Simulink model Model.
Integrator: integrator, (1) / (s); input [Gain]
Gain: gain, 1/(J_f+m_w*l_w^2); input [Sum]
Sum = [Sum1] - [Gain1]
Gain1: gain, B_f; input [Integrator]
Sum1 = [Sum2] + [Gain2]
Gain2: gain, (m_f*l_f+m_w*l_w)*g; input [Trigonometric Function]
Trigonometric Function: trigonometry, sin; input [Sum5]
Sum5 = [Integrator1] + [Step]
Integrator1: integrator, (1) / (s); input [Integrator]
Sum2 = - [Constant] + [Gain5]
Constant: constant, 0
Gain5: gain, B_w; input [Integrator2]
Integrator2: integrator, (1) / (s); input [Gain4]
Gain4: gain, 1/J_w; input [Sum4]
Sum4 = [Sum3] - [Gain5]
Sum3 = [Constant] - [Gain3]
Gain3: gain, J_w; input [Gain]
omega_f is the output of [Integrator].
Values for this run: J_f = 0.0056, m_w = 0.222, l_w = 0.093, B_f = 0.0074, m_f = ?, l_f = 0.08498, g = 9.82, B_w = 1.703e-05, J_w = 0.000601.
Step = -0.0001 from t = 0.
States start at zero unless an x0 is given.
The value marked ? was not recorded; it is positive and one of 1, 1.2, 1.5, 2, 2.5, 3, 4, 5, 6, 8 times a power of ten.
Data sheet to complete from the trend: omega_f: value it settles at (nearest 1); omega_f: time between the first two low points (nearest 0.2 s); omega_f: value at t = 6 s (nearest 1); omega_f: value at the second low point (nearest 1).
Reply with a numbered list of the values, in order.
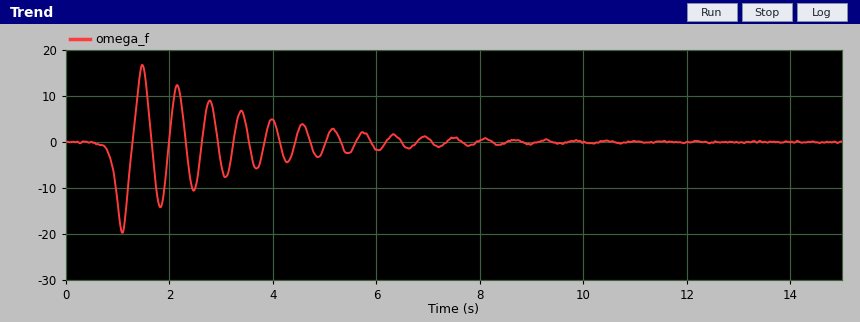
1. 0
2. 0.8 s
3. -2
4. -14
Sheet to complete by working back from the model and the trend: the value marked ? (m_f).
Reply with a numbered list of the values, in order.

1. 0.8
